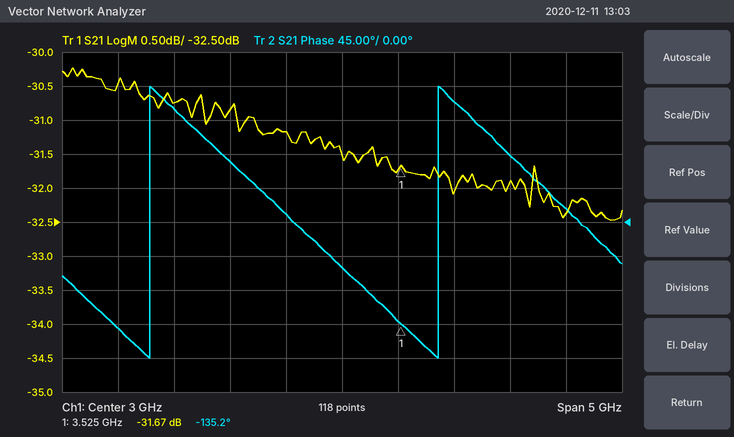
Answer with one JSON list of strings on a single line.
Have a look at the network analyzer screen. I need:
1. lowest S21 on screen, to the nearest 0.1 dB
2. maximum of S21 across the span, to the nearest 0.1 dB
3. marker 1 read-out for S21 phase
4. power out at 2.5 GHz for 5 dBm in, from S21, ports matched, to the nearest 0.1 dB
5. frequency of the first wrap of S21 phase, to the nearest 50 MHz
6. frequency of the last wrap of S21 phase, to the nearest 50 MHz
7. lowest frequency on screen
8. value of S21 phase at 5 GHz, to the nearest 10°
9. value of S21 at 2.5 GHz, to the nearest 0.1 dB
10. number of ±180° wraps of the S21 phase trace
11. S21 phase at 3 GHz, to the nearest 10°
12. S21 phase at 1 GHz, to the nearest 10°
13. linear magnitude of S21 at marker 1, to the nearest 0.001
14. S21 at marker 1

["-32.5 dB", "-30.2 dB", "-135.2°", "-26.2 dBm", "1.30 GHz", "3.85 GHz", "500 MHz", "20°", "-31.2 dB", "2", "-60°", "-140°", "0.026", "-31.67 dB"]
